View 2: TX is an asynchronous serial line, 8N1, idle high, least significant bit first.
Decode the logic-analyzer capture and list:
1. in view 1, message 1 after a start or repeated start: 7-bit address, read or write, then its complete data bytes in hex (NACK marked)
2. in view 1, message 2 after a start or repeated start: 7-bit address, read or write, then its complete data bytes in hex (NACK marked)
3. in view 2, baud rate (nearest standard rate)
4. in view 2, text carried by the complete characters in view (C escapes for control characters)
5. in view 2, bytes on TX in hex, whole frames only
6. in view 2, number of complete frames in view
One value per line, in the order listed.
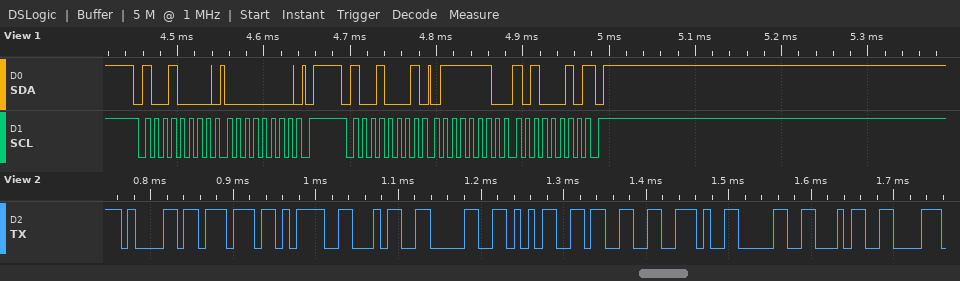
0x48 write: 00
0x48 read: 7E A2 NACK
115200 baud
"aw=4053.04"
61 77 3D 34 30 35 33 2E 30 34
10
